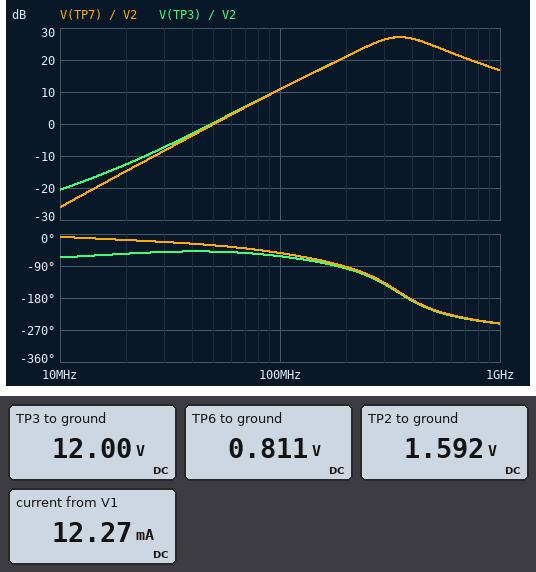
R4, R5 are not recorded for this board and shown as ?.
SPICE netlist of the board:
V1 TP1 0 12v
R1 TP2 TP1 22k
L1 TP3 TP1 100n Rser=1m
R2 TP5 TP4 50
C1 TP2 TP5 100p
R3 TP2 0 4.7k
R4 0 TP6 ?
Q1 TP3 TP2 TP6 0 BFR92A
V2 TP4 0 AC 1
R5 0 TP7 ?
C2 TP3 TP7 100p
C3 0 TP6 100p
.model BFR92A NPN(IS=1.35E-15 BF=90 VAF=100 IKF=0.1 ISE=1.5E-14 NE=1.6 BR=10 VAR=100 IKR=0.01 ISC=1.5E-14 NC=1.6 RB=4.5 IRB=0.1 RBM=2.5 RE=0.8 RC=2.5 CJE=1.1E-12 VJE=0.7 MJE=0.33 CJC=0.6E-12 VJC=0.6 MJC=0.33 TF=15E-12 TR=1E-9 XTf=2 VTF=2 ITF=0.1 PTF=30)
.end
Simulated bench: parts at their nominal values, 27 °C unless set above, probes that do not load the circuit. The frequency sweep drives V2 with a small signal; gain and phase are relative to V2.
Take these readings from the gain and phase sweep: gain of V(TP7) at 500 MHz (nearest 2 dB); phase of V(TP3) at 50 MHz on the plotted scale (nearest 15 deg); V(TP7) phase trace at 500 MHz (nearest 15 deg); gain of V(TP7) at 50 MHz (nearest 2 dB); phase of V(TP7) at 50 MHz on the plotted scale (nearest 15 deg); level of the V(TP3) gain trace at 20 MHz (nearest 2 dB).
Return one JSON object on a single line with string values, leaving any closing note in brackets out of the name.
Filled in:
{"gain of V(TP7) at 500 MHz": "24 dB", "phase of V(TP3) at 50 MHz on the plotted scale": "-45 deg", "V(TP7) phase trace at 500 MHz": "-210 deg", "gain of V(TP7) at 50 MHz": "0 dB", "phase of V(TP7) at 50 MHz on the plotted scale": "-30 deg", "level of the V(TP3) gain trace at 20 MHz": "-12 dB"}
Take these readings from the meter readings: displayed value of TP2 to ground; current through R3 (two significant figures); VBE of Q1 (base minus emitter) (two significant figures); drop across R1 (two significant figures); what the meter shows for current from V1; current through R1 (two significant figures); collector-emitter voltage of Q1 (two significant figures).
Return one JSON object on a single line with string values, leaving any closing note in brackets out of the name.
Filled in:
{"displayed value of TP2 to ground": "1.592 V", "current through R3": "340 µA", "VBE of Q1 (base minus emitter)": "780 mV", "drop across R1": "10 V", "what the meter shows for current from V1": "12.27 mA", "current through R1": "470 µA", "collector-emitter voltage of Q1": "11 V"}
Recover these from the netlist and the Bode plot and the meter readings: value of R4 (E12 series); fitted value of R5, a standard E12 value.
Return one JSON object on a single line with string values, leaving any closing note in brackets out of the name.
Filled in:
{"value of R4": "68 Ω", "fitted value of R5, a standard E12 value": "100 Ω"}
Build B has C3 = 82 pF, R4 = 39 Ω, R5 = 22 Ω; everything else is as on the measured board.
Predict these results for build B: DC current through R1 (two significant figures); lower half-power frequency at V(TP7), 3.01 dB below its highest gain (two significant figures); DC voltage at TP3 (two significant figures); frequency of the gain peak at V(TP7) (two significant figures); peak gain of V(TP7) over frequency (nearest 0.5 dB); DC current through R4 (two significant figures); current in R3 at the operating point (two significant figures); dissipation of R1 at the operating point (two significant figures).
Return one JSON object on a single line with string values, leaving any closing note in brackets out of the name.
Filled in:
{"DC current through R1": "480 µA", "lower half-power frequency at V(TP7), 3.01 dB below its highest gain": "300 MHz", "DC voltage at TP3": "12 V", "frequency of the gain peak at V(TP7)": "500 MHz", "peak gain of V(TP7) over frequency": "14.0 dB", "DC current through R4": "16 mA", "current in R3 at the operating point": "300 µA", "dissipation of R1 at the operating point": "5.1 mW"}
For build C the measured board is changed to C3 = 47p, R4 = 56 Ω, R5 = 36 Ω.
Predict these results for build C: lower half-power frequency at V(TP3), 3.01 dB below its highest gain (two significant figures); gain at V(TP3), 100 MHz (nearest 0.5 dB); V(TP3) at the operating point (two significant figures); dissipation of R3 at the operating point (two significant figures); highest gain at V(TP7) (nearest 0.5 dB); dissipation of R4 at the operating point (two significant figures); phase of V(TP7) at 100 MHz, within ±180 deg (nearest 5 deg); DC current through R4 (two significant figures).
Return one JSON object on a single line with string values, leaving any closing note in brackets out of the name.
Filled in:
{"lower half-power frequency at V(TP3), 3.01 dB below its highest gain": "400 MHz", "gain at V(TP3), 100 MHz": "2.5 dB", "V(TP3) at the operating point": "12 V", "dissipation of R3 at the operating point": "500 µW", "highest gain at V(TP7)": "17.0 dB", "dissipation of R4 at the operating point": "9.9 mW", "phase of V(TP7) at 100 MHz, within ±180 deg": "-90 deg", "DC current through R4": "13 mA"}
